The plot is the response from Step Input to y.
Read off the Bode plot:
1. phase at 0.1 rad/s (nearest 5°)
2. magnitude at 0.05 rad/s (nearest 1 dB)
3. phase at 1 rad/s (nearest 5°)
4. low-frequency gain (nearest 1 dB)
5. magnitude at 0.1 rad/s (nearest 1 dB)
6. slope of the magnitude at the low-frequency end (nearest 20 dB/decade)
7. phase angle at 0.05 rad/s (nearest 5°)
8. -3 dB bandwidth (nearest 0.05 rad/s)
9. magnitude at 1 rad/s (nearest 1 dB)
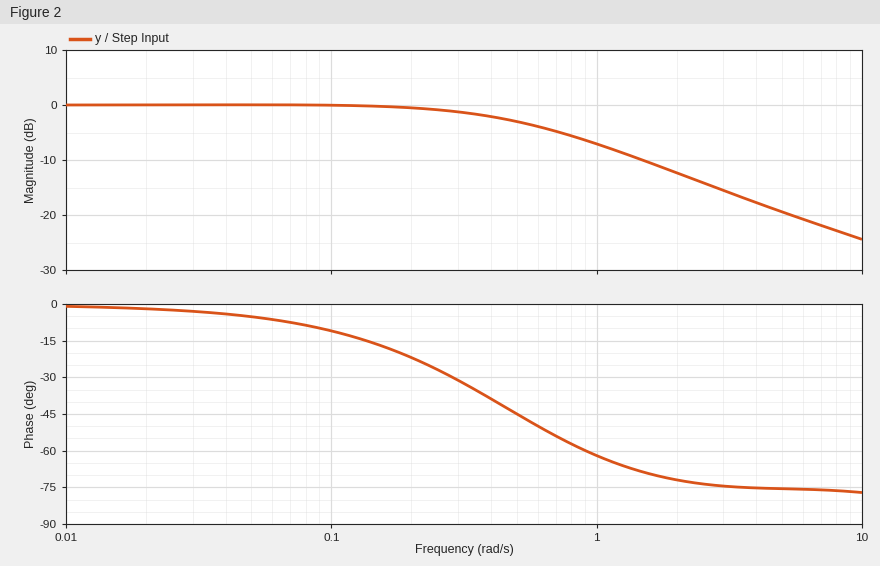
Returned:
-10°
0 dB
-60°
0 dB
0 dB
0 dB/decade
-5°
0.50 rad/s
-7 dB
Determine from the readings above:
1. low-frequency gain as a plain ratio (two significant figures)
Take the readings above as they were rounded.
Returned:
1.0
